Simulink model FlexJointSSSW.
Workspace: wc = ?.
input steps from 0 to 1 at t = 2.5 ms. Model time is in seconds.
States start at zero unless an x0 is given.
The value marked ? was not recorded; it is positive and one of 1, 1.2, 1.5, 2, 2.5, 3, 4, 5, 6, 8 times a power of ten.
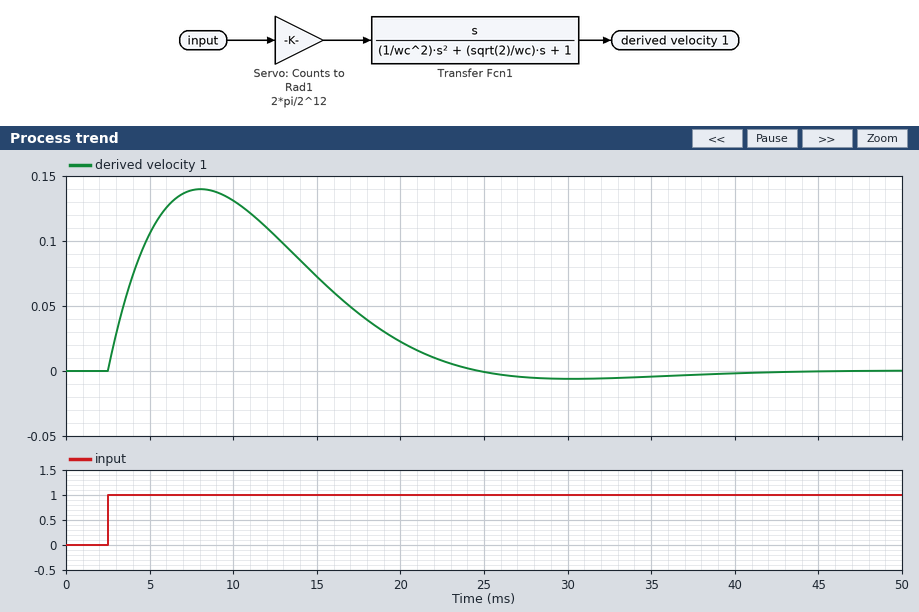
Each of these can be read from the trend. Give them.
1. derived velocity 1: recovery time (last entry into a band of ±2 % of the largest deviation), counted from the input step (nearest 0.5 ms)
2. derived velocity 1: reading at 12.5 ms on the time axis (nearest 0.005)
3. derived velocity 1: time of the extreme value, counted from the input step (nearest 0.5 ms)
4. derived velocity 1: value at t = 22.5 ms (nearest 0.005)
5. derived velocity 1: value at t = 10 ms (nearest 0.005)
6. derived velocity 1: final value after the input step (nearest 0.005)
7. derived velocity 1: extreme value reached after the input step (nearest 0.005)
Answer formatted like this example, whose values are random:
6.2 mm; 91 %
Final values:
35.5 ms; 0.105; 5.5 ms; 0.010; 0.130; 0.000; 0.140
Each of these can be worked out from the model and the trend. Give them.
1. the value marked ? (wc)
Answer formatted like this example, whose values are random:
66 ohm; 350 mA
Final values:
200
